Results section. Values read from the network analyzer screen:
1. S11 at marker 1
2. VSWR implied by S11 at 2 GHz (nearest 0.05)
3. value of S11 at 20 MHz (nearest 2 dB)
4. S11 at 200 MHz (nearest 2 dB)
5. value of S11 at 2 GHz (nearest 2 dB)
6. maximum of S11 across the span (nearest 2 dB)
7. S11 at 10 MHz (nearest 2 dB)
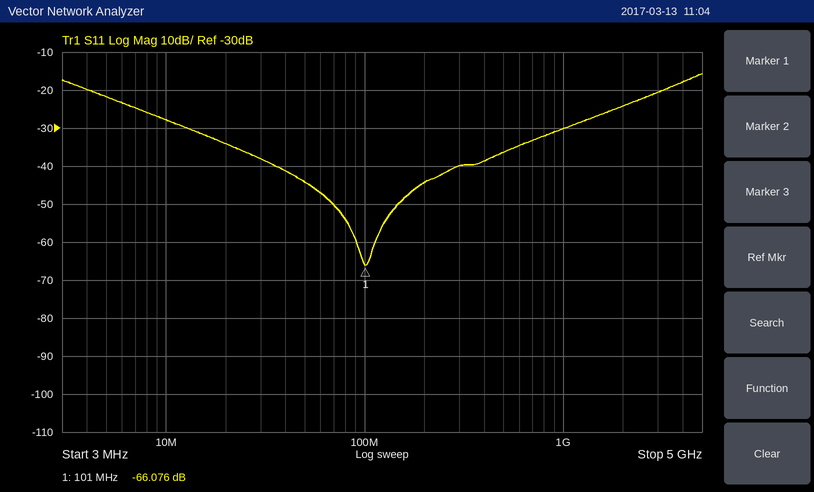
-66.076 dB
1.15
-34 dB
-44 dB
-24 dB
-16 dB
-28 dB
